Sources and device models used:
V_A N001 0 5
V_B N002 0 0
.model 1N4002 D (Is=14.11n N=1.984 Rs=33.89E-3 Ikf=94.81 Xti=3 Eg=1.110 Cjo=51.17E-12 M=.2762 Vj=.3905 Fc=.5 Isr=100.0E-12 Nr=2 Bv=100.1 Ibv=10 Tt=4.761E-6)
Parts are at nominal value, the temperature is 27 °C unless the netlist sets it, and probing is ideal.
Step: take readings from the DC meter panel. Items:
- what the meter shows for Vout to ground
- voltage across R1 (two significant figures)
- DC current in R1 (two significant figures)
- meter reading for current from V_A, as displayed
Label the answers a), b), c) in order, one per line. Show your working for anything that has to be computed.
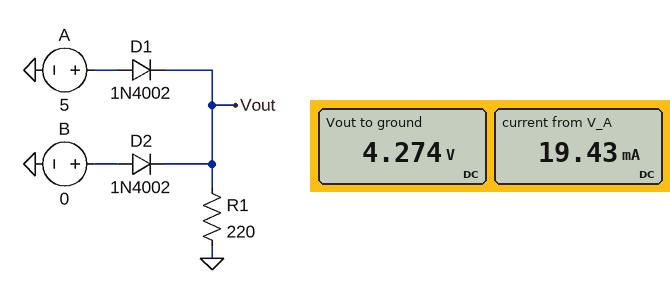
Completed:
a) 4.274 V
b) 4.274 V = 4.3 V
c) (4.274 V) / 220 Ω = 19 mA
d) 19.43 mA
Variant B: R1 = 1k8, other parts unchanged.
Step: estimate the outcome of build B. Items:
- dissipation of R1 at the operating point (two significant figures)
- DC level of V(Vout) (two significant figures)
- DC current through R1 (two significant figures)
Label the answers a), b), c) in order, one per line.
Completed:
a) 11 mW
b) 4.4 V
c) 2.4 mA
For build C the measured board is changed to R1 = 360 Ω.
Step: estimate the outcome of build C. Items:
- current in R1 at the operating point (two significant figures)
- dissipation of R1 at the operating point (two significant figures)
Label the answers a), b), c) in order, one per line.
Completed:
a) 12 mA
b) 51 mW
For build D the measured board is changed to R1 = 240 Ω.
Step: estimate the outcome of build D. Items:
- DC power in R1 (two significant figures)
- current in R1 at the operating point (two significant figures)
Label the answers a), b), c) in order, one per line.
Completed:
a) 76 mW
b) 18 mA
